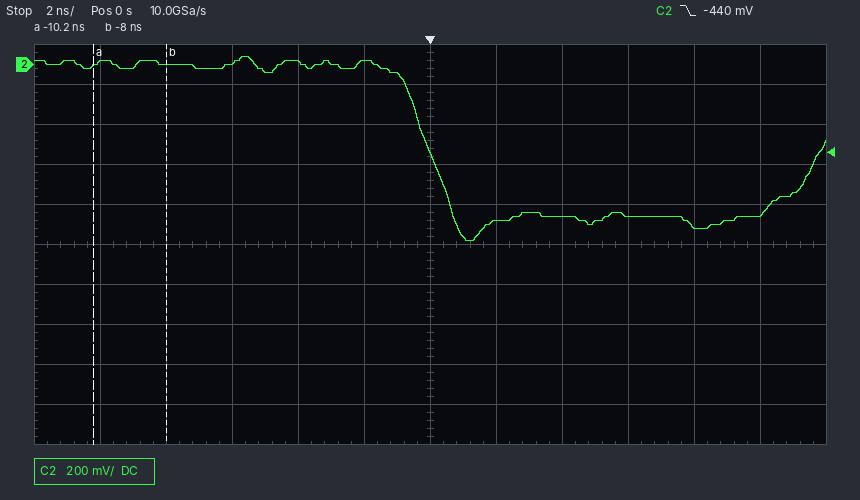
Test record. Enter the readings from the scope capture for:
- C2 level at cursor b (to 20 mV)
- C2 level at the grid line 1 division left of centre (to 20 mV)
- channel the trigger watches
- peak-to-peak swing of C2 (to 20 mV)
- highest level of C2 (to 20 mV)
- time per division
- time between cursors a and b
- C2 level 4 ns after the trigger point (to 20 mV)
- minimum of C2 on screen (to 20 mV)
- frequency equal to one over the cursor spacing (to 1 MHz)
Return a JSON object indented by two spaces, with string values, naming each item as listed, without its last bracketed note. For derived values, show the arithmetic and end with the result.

{
  "C2 level at cursor b": "0 mV",
  "C2 level at the grid line 1 division left of centre": "20 mV",
  "channel the trigger watches": "C2",
  "peak-to-peak swing of C2": "40 mV − (-880 mV) = 920 mV",
  "highest level of C2": "40 mV",
  "time per division": "2 ns",
  "time between cursors a and b": "-8 ns − (-10.2 ns) = 2.2 ns",
  "C2 level 4 ns after the trigger point": "-760 mV",
  "minimum of C2 on screen": "-880 mV",
  "frequency equal to one over the cursor spacing": "1 / 2.2 ns ≈ 455 MHz"
}
